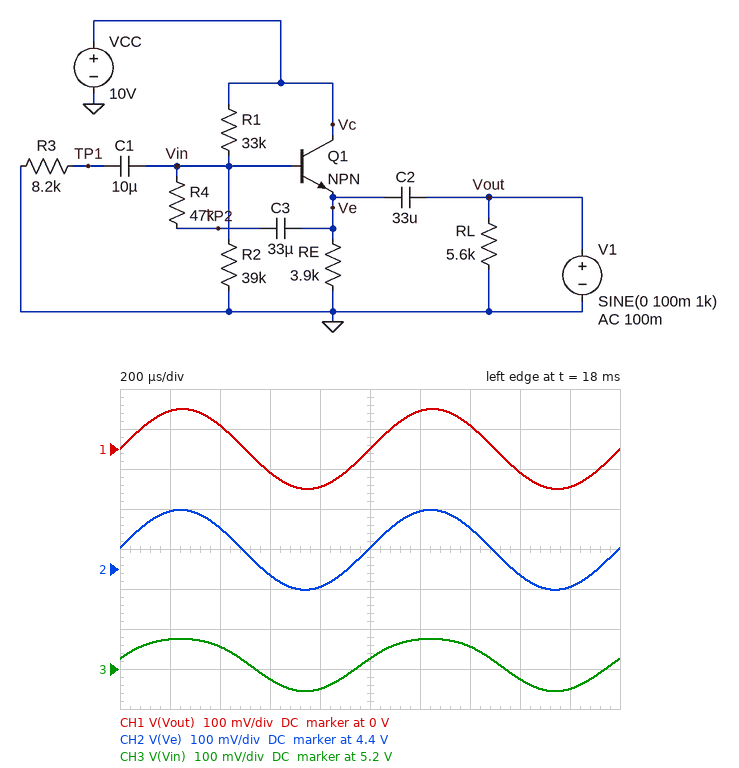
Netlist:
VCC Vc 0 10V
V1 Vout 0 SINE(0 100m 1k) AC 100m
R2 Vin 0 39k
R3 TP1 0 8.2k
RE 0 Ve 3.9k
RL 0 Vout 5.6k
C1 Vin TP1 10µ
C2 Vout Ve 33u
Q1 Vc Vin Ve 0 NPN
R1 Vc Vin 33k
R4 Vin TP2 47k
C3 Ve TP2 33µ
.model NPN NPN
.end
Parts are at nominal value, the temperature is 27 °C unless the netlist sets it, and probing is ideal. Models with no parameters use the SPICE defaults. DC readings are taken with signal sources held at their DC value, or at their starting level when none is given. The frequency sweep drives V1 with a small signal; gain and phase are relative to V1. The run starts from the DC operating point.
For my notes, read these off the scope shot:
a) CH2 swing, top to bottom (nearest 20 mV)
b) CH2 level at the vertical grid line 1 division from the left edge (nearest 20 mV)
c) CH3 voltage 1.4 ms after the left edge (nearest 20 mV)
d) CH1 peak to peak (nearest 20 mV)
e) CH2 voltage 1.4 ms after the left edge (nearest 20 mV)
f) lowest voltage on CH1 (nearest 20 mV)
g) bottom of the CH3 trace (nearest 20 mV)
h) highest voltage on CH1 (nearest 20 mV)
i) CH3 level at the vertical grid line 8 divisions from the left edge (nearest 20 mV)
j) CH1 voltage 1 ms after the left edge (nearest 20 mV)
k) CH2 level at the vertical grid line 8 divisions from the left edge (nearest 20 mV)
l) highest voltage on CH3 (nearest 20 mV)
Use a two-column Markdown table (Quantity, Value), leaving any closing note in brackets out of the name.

| Quantity | Value |
|---|---|
| CH2 swing, top to bottom | 200 mV |
| CH2 level at the vertical grid line 1 division from the left edge | 4.54 V |
| CH3 voltage 1.4 ms after the left edge | 5.26 V |
| CH1 peak to peak | 200 mV |
| CH2 voltage 1.4 ms after the left edge | 4.50 V |
| lowest voltage on CH1 | -100 mV |
| bottom of the CH3 trace | 5.14 V |
| highest voltage on CH1 | 100 mV |
| CH3 level at the vertical grid line 8 divisions from the left edge | 5.18 V |
| CH1 voltage 1 ms after the left edge | 0 V |
| CH2 level at the vertical grid line 8 divisions from the left edge | 4.38 V |
| highest voltage on CH3 | 5.28 V |
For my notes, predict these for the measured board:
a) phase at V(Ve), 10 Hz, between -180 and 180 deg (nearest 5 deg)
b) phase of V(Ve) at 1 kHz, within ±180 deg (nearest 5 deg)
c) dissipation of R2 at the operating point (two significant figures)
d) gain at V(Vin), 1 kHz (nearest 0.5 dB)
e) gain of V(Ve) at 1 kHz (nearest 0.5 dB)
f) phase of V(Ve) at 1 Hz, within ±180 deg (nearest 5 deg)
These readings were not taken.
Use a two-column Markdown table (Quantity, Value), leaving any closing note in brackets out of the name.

| Quantity | Value |
|---|---|
| phase at V(Ve), 10 Hz, between -180 and 180 deg | 75 deg |
| phase of V(Ve) at 1 kHz, within ±180 deg | 5 deg |
| dissipation of R2 at the operating point | 700 µW |
| gain at V(Vin), 1 kHz | -3.0 dB |
| gain of V(Ve) at 1 kHz | 0 dB |
| phase of V(Ve) at 1 Hz, within ±180 deg | 65 deg |
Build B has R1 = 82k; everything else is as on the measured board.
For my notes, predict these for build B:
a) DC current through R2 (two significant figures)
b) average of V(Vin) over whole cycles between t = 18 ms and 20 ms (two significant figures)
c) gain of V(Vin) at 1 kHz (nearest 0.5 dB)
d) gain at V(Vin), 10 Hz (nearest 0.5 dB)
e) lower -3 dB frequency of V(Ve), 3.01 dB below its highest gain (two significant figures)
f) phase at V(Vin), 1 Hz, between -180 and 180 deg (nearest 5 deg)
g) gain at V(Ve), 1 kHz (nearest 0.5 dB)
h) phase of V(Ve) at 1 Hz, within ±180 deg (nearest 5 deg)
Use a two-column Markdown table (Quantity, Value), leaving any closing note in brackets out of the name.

| Quantity | Value |
|---|---|
| DC current through R2 | 79 µA |
| average of V(Vin) over whole cycles between t = 18 ms and 20 ms | 3.1 V |
| gain of V(Vin) at 1 kHz | -4.5 dB |
| gain at V(Vin), 10 Hz | -17.5 dB |
| lower -3 dB frequency of V(Ve), 3.01 dB below its highest gain | 45 Hz |
| phase at V(Vin), 1 Hz, between -180 and 180 deg | 50 deg |
| gain at V(Ve), 1 kHz | 0 dB |
| phase of V(Ve) at 1 Hz, within ±180 deg | 60 deg |
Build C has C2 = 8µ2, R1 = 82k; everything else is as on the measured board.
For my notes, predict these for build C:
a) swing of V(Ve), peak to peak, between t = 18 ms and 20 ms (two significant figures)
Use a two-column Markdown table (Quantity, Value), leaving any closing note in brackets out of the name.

| Quantity | Value |
|---|---|
| swing of V(Ve), peak to peak, between t = 18 ms and 20 ms | 200 mV |
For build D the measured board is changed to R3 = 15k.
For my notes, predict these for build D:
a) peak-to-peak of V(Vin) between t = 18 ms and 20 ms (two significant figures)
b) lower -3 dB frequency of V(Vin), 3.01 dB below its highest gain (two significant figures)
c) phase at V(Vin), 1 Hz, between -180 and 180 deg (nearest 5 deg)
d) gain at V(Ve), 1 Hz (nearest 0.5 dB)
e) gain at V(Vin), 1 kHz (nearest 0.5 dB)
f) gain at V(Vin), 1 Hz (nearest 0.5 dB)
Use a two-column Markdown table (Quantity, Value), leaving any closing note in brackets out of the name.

| Quantity | Value |
|---|---|
| peak-to-peak of V(Vin) between t = 18 ms and 20 ms | 150 mV |
| lower -3 dB frequency of V(Vin), 3.01 dB below its highest gain | 47 Hz |
| phase at V(Vin), 1 Hz, between -180 and 180 deg | 70 deg |
| gain at V(Ve), 1 Hz | -31.5 dB |
| gain at V(Vin), 1 kHz | -2.0 dB |
| gain at V(Vin), 1 Hz | -33.0 dB |
